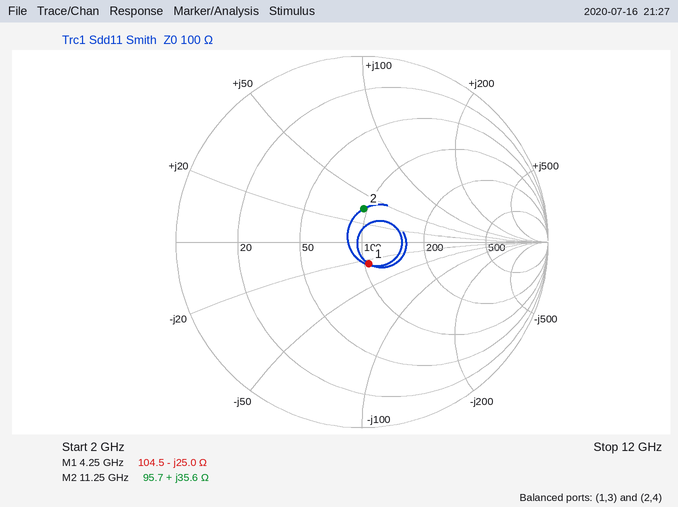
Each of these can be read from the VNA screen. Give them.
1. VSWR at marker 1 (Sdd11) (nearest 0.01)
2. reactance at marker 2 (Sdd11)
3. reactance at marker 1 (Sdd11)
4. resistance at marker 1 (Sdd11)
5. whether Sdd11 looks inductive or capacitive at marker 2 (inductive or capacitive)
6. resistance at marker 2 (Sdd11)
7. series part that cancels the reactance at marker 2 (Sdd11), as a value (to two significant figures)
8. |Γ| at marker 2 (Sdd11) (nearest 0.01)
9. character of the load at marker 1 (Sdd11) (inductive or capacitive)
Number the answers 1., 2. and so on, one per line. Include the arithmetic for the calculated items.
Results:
1. 1.28
2. +35.6 Ω
3. -25.0 Ω
4. 104.5 Ω
5. inductive
6. 95.7 Ω
7. C = 1/(2π × 11.25 GHz × 35.6 Ω) ≈ 397 fF, so 400 fF to two significant figures
8. 0.18
9. capacitive
